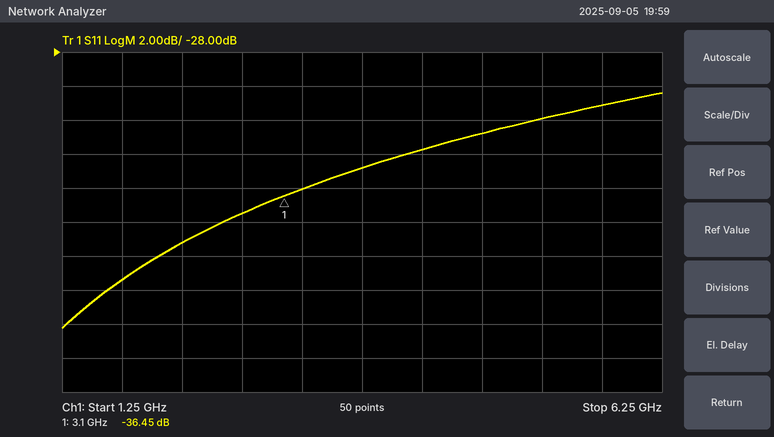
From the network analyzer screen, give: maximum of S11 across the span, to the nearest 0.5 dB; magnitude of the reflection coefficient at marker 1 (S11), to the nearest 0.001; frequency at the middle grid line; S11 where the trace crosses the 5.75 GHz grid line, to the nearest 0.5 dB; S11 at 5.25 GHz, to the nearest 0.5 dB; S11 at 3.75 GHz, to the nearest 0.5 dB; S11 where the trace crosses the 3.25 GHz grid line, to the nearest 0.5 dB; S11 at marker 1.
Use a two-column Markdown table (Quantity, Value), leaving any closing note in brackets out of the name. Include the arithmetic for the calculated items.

| Quantity | Value |
|---|---|
| maximum of S11 across the span, to the nearest 0.5 dB | -30.5 dB |
| magnitude of the reflection coefficient at marker 1 (S11), to the nearest 0.001 | 10^(-36.45/20) ≈ 0.015 |
| frequency at the middle grid line | 3.75 GHz |
| S11 where the trace crosses the 5.75 GHz grid line, to the nearest 0.5 dB | -31.0 dB |
| S11 at 5.25 GHz, to the nearest 0.5 dB | -32.0 dB |
| S11 at 3.75 GHz, to the nearest 0.5 dB | -35.0 dB |
| S11 where the trace crosses the 3.25 GHz grid line, to the nearest 0.5 dB | -36.0 dB |
| S11 at marker 1 | -36.45 dB |
